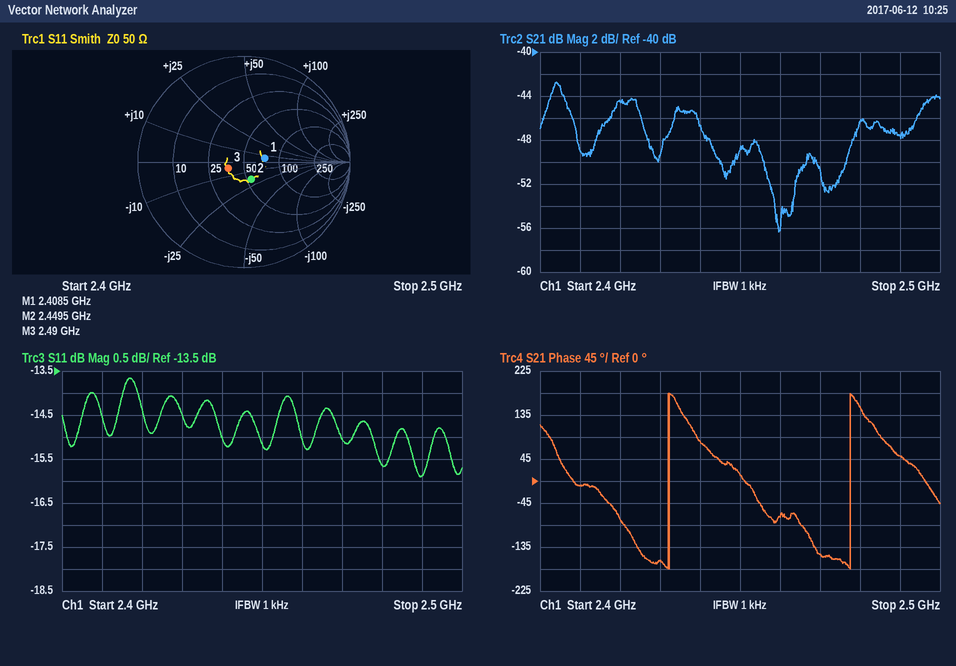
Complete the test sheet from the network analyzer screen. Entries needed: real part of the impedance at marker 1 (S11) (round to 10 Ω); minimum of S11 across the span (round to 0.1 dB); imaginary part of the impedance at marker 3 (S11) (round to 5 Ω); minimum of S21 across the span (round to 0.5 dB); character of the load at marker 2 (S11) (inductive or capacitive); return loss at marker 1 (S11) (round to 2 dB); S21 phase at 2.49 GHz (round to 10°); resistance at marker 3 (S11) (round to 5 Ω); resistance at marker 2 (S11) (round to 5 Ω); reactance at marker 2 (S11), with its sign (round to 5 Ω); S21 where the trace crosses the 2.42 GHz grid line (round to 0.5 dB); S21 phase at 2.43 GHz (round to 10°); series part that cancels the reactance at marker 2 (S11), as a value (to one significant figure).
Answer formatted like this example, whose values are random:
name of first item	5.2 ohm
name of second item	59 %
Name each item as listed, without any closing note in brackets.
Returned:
real part of the impedance at marker 1 (S11)	70 Ω
minimum of S11 across the span	-15.9 dB
imaginary part of the impedance at marker 3 (S11)	-5 Ω
minimum of S21 across the span	-56.5 dB
character of the load at marker 2 (S11)	capacitive
return loss at marker 1 (S11)	14 dB
S21 phase at 2.49 GHz	50°
resistance at marker 3 (S11)	35 Ω
resistance at marker 2 (S11)	55 Ω
reactance at marker 2 (S11), with its sign	-20 Ω
S21 where the trace crosses the 2.42 GHz grid line	-44.5 dB
S21 phase at 2.43 GHz	-160°
series part that cancels the reactance at marker 2 (S11), as a value	1 nH
